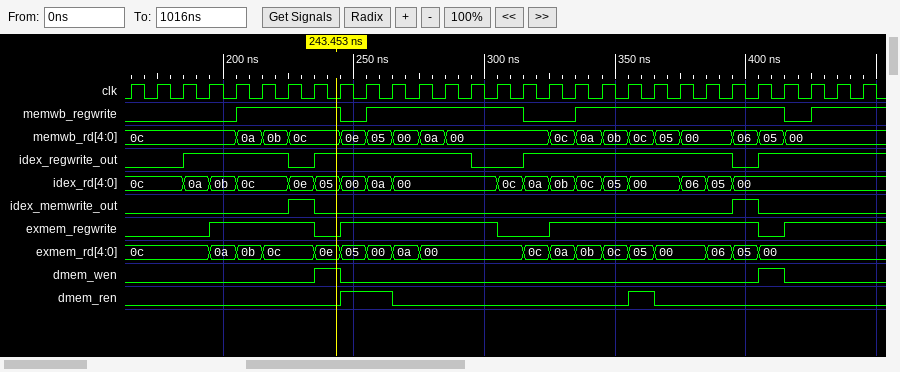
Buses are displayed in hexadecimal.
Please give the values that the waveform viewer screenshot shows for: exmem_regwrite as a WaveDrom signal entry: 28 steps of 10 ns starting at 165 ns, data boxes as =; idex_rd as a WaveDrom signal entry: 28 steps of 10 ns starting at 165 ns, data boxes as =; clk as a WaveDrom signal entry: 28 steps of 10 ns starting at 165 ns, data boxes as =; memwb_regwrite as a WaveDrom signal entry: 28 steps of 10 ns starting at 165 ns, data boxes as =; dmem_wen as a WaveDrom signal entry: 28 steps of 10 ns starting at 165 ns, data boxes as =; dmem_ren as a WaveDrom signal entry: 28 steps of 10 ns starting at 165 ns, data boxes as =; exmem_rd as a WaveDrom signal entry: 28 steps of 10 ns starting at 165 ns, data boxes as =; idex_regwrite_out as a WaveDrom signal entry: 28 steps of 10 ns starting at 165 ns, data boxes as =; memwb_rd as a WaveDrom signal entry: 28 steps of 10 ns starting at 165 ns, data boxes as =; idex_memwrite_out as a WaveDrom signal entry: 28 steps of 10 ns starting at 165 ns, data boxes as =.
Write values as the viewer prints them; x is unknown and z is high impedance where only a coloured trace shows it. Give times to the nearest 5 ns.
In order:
{name: 'exmem_regwrite', wave: '0..1...01.....0.1.......01..'}
{name: 'idex_rd', wave: '=.===.=====...======.===....', data: '0c 0a 0b 0c 0e 05 00 0a 00 0c 0a 0b 0c 05 00 06 05 00'}
{name: 'clk', wave: 'p...........................'}
{name: 'memwb_regwrite', wave: '0...1...01.....0.1.......01.'}
{name: 'dmem_wen', wave: '0......10...............10..'}
{name: 'dmem_ren', wave: '0.......1.0........10.......'}
{name: 'exmem_rd', wave: '=..===.=====...======.===...', data: '0c 0a 0b 0c 0e 05 00 0a 00 0c 0a 0b 0c 05 00 06 05 00'}
{name: 'idex_regwrite_out', wave: '0.1...01.....0.1.......01...'}
{name: 'memwb_rd', wave: '=...===.=====...======.===..', data: '0c 0a 0b 0c 0e 05 00 0a 00 0c 0a 0b 0c 05 00 06 05 00'}
{name: 'idex_memwrite_out', wave: '0.....10...............10...'}
